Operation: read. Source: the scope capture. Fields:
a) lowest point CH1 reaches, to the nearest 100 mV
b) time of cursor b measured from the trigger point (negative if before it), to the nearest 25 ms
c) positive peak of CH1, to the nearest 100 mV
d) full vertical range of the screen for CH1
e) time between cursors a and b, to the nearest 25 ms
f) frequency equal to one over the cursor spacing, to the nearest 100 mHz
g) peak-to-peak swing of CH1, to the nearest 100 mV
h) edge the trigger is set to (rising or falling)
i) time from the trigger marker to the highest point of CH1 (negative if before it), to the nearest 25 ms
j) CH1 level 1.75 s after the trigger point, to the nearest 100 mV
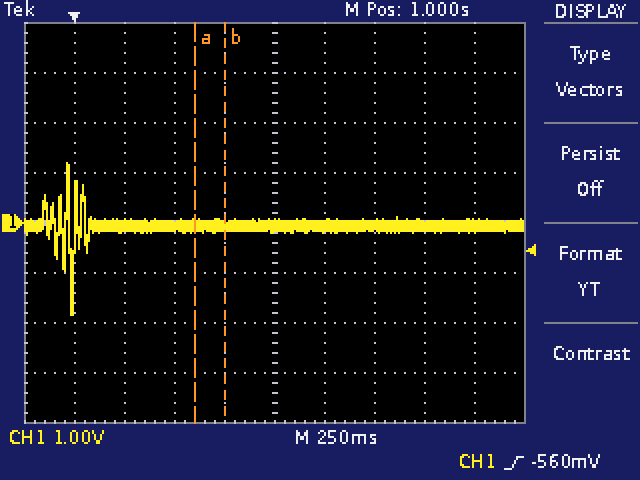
-1.8 V
+750 ms
1.2 V
8 V
150 ms
6.7 Hz
3.0 V
rising
-25 ms
-100 mV
